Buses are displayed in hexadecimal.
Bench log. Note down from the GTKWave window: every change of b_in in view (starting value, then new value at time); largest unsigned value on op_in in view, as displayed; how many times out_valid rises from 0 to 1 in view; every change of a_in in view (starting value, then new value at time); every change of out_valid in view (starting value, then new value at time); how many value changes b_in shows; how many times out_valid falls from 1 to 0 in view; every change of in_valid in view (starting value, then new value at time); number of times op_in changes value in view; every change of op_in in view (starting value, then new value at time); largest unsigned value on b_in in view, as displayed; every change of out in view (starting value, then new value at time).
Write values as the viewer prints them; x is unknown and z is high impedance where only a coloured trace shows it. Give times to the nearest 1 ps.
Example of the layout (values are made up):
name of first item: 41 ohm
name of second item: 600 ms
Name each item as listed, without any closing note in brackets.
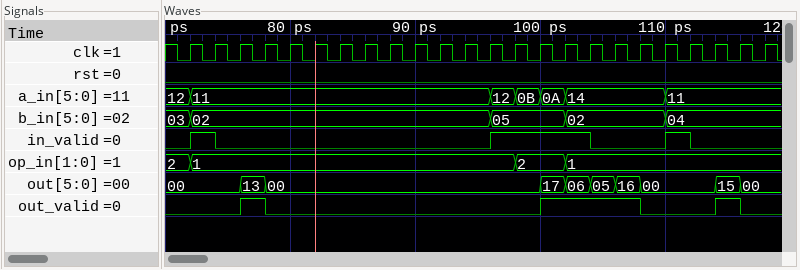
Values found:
every change of b_in in view: 03, 02 at 72 ps, 05 at 96 ps, 02 at 102 ps, 04 at 110 ps
largest unsigned value on op_in in view, as displayed: 2
how many times out_valid rises from 0 to 1 in view: 3
every change of a_in in view: 12, 11 at 72 ps, 12 at 96 ps, 0B at 98 ps, 0A at 100 ps, 14 at 102 ps, 11 at 110 ps
every change of out_valid in view: 0, 1 at 76 ps, 0 at 78 ps, 1 at 100 ps, 0 at 108 ps, 1 at 114 ps, 0 at 116 ps
how many value changes b_in shows: 4
how many times out_valid falls from 1 to 0 in view: 3
every change of in_valid in view: 0, 1 at 72 ps, 0 at 74 ps, 1 at 96 ps, 0 at 104 ps, 1 at 110 ps, 0 at 112 ps
number of times op_in changes value in view: 3
every change of op_in in view: 2, 1 at 72 ps, 2 at 98 ps, 1 at 102 ps
largest unsigned value on b_in in view, as displayed: 05
every change of out in view: 00, 13 at 76 ps, 00 at 78 ps, 17 at 100 ps, 06 at 102 ps, 05 at 104 ps, 16 at 106 ps, 00 at 108 ps, 15 at 114 ps, 00 at 116 ps
